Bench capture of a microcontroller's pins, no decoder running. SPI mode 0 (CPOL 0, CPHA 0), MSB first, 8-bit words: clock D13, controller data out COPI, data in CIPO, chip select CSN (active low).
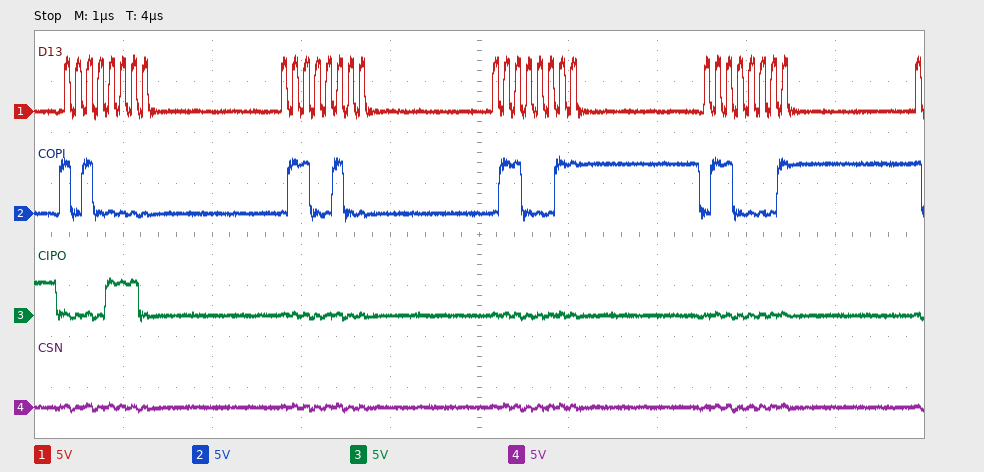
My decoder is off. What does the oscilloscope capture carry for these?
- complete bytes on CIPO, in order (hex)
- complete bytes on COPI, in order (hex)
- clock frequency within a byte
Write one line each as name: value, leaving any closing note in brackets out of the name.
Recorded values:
complete bytes on CIPO, in order: 0x0E 0x00 0x00 0x00
complete bytes on COPI, in order: 0xA0 0x64 0x63 0x61
clock frequency within a byte: 8 MHz
